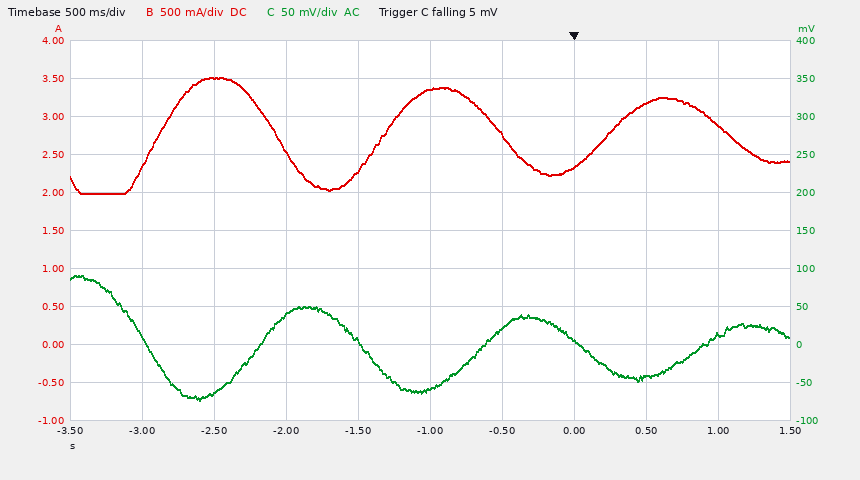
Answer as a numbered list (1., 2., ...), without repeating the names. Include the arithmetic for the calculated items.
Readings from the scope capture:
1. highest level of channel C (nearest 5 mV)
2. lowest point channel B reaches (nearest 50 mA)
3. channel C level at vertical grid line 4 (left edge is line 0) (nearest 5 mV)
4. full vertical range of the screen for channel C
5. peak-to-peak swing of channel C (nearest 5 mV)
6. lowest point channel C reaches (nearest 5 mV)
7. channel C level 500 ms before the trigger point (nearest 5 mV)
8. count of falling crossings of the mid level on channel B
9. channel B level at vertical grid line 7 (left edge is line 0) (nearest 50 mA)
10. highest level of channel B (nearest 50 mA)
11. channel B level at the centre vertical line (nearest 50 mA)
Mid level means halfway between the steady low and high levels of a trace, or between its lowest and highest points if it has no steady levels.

1. 90 mV
2. 2.00 A
3. 5 mV
4. 500 mV
5. 90 mV − (-75 mV) = 165 mV
6. -75 mV
7. 20 mV
8. 3
9. 2.35 A
10. 3.50 A
11. 3.35 A
